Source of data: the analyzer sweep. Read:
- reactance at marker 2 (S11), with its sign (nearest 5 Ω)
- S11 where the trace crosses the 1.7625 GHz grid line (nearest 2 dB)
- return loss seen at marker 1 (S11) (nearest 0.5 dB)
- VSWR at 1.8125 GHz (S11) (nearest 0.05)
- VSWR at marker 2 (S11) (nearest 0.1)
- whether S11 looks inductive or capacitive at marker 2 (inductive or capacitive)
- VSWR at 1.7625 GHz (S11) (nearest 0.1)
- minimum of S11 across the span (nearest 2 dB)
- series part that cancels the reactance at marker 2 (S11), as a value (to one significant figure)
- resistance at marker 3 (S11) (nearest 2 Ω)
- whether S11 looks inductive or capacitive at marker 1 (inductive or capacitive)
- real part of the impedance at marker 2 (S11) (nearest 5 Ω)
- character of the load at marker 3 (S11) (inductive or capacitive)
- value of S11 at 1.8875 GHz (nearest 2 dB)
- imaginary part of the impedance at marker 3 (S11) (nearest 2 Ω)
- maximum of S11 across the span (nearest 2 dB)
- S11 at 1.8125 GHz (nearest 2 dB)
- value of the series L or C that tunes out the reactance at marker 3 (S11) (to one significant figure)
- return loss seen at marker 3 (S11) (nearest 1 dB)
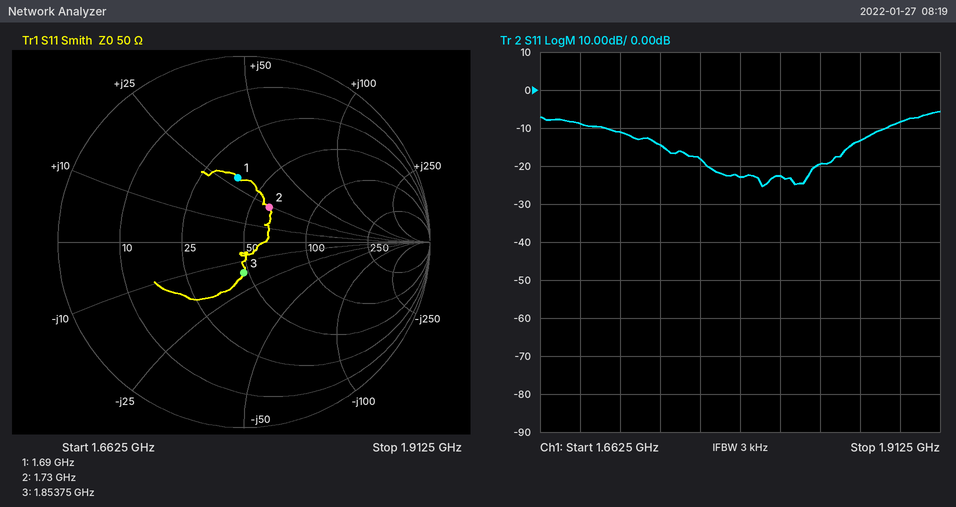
+25 Ω
-18 dB
9.0 dB
1.15
1.6
inductive
1.3
-26 dB
4 pF
48 Ω
inductive
60 Ω
capacitive
-8 dB
-16 Ω
-6 dB
-22 dB
1 nH
16 dB
